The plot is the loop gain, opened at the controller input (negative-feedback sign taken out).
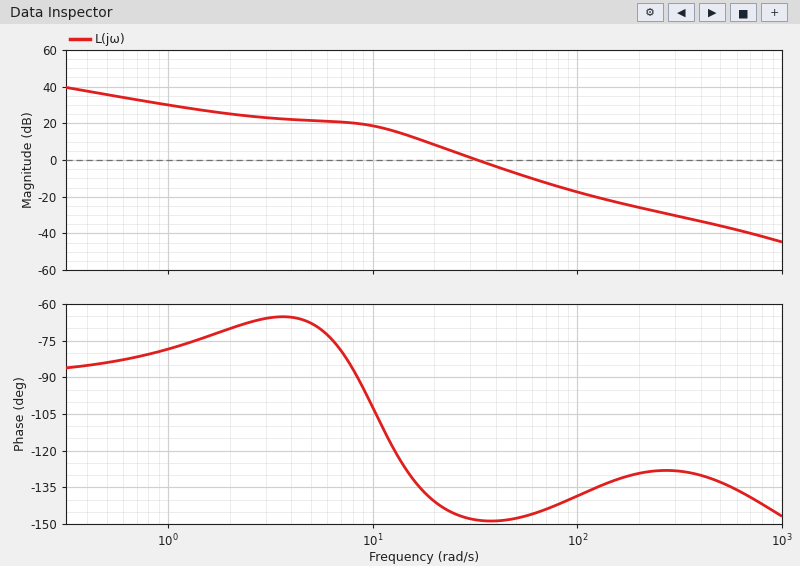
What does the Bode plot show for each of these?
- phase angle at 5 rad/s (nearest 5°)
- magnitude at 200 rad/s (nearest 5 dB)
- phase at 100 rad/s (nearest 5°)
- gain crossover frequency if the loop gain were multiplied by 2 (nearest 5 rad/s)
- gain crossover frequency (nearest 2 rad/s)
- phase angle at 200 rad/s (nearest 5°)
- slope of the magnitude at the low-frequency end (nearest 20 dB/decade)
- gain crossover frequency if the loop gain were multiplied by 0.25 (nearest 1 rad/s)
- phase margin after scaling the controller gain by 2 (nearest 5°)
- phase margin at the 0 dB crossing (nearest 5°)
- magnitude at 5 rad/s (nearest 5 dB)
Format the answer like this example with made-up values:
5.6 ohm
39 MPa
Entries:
-70°
-25 dB
-140°
45 rad/s
32 rad/s
-130°
-20 dB/decade
16 rad/s
30°
30°
20 dB
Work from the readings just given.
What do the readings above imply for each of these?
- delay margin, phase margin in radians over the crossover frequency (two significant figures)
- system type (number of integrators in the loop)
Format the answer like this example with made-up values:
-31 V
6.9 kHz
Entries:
0.016 s
1
